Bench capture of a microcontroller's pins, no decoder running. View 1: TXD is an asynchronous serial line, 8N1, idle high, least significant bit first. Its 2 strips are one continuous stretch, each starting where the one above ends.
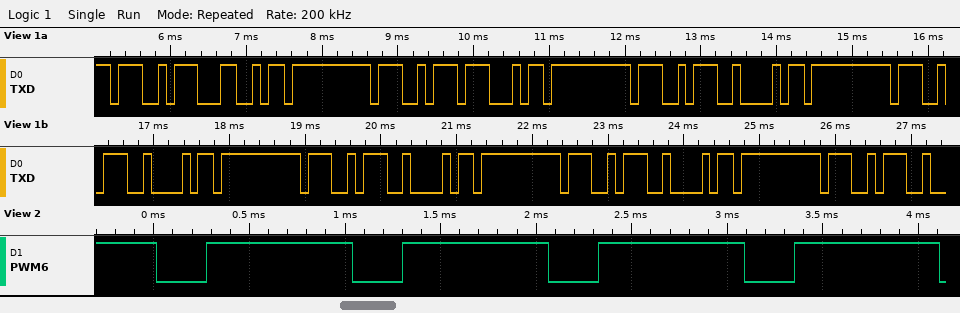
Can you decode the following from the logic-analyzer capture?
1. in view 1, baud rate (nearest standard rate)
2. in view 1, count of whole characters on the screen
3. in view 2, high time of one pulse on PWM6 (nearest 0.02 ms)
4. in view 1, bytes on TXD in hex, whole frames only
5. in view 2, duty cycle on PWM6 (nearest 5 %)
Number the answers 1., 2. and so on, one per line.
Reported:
1. 9600 baud
2. 19
3. 0.76 ms
4. A7 4C FF A7 47 FF A7 42 FF A7 42 FF A7 42 FF A7 42 FF A7
5. 75 %
